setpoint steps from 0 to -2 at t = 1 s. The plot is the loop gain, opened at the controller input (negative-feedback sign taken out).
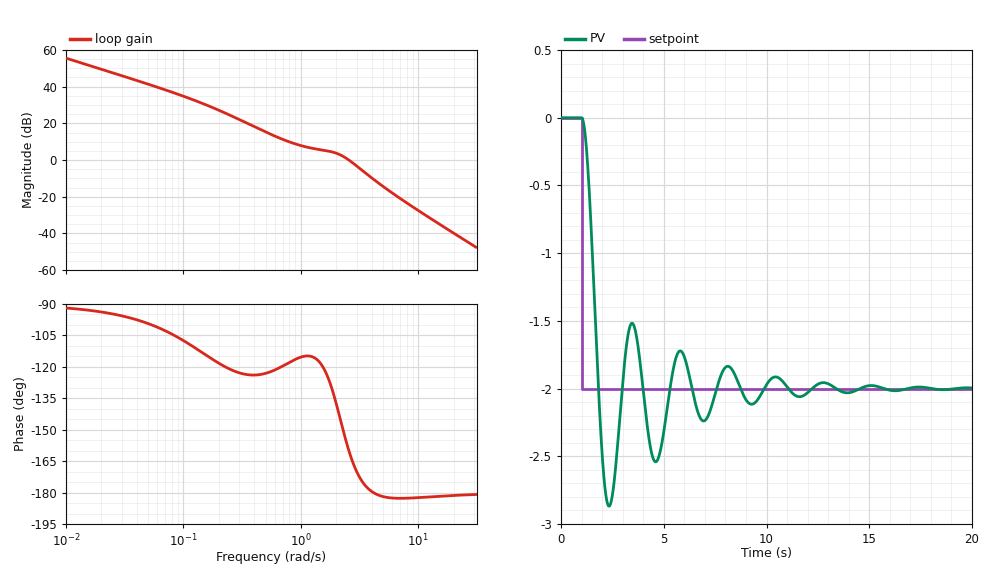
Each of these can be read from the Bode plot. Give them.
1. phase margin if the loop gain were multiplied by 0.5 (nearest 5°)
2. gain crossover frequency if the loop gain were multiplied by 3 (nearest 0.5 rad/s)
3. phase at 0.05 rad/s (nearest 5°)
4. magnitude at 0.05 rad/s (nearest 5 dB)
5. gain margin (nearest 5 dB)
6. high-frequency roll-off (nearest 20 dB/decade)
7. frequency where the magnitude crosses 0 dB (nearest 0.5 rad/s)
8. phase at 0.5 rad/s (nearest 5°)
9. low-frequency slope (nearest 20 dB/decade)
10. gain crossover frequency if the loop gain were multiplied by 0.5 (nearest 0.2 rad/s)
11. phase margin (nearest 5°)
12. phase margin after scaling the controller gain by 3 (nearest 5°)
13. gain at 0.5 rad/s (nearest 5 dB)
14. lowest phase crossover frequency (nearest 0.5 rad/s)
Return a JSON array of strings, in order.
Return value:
["65°", "4.0 rad/s", "-100°", "40 dB", "10 dB", "-40 dB/decade", "2.5 rad/s", "-125°", "-20 dB/decade", "1.4 rad/s", "20°", "0°", "15 dB", "4.0 rad/s"]
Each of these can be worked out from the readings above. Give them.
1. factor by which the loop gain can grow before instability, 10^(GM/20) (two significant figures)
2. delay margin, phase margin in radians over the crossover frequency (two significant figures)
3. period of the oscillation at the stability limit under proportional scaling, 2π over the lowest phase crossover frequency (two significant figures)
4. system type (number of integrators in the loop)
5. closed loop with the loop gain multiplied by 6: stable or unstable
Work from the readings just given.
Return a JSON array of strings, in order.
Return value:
["3.2", "0.14 s", "1.6 s", "1", "unstable"]
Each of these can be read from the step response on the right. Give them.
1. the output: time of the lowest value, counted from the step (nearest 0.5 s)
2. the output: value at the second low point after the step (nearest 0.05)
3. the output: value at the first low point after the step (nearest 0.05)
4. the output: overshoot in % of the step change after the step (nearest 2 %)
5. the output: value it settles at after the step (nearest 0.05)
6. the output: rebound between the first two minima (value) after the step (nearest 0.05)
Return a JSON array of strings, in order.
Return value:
["1.5 s", "-2.55", "-2.85", "44 %", "-2.00", "-1.50"]
